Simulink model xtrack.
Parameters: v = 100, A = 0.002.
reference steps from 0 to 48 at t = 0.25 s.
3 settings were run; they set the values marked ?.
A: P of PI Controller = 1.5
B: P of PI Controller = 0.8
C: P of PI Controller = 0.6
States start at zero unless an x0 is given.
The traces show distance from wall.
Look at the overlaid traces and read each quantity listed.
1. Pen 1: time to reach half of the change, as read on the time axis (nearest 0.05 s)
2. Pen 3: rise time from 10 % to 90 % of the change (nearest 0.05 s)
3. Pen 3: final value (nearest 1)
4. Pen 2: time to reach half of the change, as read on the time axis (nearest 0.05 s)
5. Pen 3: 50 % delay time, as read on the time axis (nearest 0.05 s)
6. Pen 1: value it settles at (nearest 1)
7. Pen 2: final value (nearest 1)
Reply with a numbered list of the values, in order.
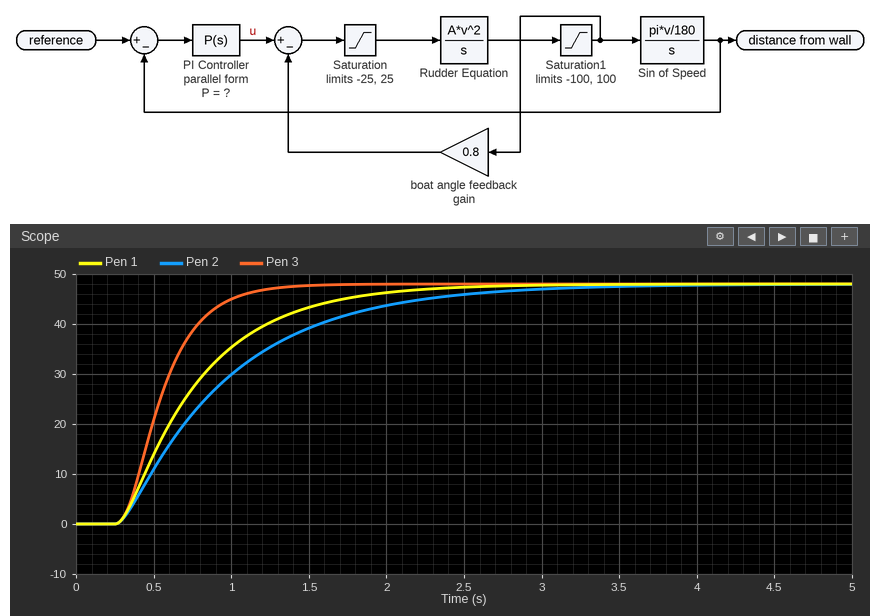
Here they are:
1. 0.70 s
2. 0.55 s
3. 48
4. 0.80 s
5. 0.55 s
6. 48
7. 48
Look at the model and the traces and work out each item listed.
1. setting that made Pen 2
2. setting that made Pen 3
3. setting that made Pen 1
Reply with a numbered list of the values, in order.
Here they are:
1. C
2. A
3. B
